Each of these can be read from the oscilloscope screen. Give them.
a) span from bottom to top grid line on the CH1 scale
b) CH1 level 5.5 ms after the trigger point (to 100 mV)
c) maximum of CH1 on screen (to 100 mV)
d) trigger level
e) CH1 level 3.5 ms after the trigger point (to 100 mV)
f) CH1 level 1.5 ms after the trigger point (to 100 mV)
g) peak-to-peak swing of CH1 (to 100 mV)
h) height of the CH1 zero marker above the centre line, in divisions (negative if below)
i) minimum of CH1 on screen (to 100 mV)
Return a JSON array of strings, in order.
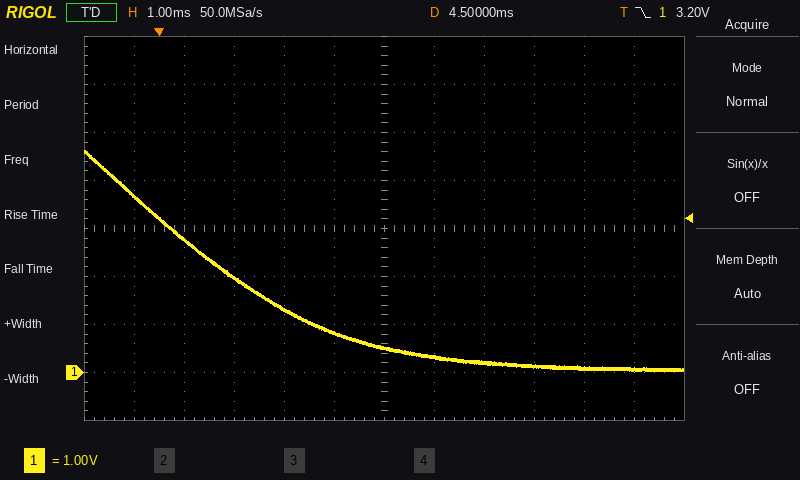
["8 V", "300 mV", "4.6 V", "3.20 V", "800 mV", "2.0 V", "4.6 V", "-3.0 div", "0.0 V"]
